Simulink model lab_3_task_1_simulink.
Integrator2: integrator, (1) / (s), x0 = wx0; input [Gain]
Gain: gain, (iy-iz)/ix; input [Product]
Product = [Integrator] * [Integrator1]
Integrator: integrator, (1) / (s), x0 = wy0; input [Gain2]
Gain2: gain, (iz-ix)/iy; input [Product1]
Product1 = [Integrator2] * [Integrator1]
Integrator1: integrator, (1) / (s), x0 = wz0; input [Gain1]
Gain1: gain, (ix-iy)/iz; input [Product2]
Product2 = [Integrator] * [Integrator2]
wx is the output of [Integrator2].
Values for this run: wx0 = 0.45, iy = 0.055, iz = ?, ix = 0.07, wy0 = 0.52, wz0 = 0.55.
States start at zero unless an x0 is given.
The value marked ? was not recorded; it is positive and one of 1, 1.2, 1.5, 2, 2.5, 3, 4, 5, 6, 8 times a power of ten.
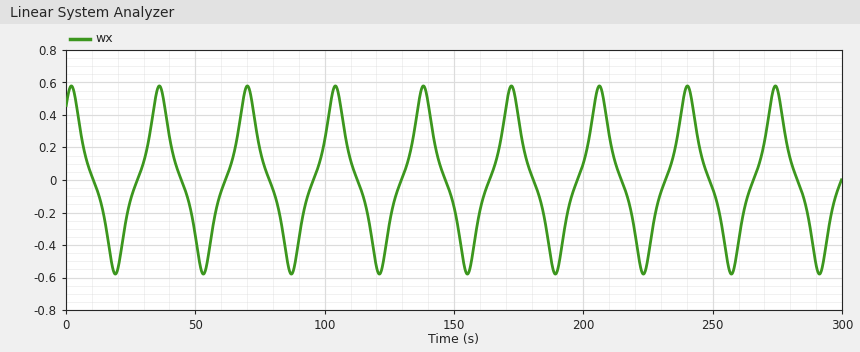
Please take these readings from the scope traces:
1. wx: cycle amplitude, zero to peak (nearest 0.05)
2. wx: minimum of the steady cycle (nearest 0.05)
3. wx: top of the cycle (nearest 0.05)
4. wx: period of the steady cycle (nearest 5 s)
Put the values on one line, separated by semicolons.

0.60; -0.60; 0.60; 35 s
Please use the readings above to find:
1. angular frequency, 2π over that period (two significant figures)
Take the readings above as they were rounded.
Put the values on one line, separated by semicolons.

0.18 rad/s
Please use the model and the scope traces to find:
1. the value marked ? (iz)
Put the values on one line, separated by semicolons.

0.03
